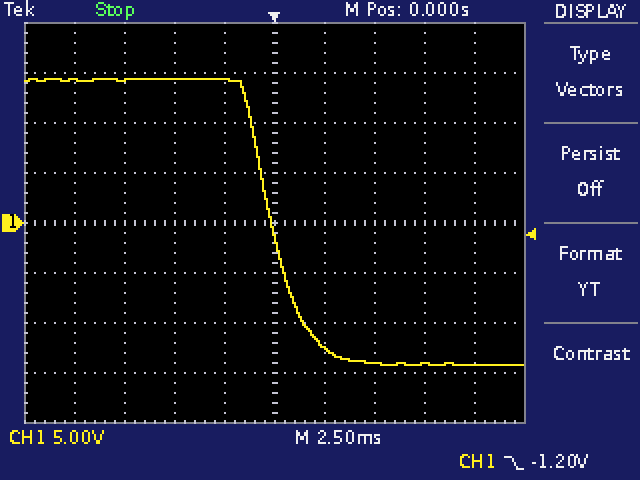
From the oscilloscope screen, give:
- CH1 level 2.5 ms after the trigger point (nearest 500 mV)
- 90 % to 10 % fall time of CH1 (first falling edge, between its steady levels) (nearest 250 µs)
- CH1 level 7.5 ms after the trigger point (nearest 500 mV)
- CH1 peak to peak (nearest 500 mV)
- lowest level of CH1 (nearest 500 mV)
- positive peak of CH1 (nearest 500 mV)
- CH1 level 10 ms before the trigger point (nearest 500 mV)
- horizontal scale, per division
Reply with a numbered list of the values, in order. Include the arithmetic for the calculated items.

1. -12.5 V
2. 3.25 ms
3. -14.0 V
4. 14.5 V − (-14.0 V) = 28.5 V
5. -14.0 V
6. 14.5 V
7. 14.5 V
8. 2.5 ms
